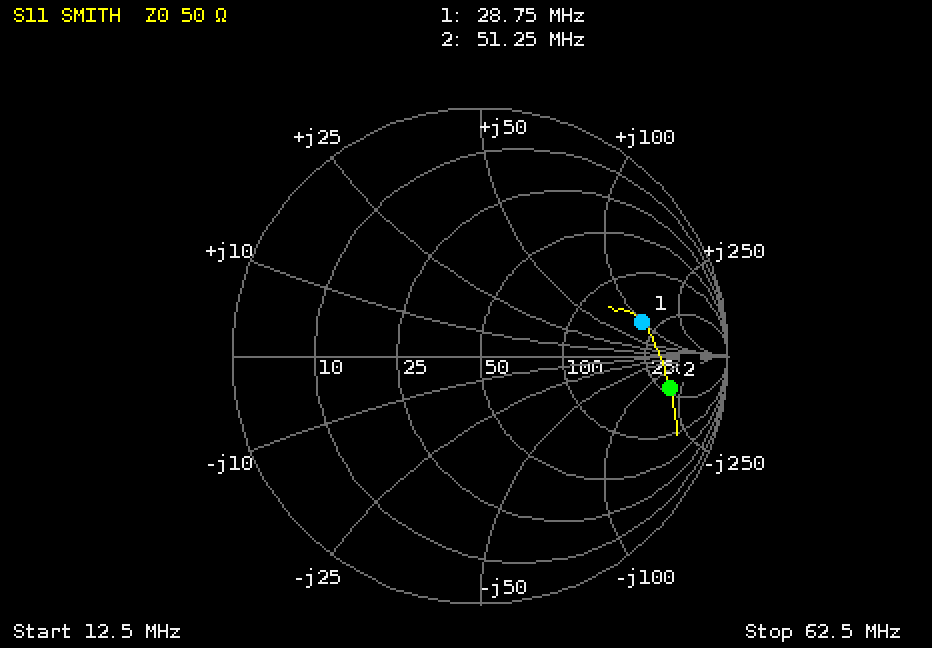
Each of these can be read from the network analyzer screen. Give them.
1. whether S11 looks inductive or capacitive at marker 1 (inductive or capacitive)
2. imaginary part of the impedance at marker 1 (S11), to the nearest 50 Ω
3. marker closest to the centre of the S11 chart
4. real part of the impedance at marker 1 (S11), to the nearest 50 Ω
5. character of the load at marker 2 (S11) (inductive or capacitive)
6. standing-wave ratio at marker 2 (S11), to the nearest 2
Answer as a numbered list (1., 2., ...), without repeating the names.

1. inductive
2. +100 Ω
3. marker 1
4. 200 Ω
5. capacitive
6. 8
